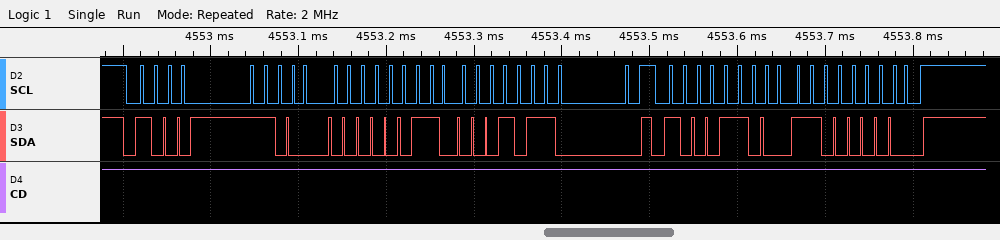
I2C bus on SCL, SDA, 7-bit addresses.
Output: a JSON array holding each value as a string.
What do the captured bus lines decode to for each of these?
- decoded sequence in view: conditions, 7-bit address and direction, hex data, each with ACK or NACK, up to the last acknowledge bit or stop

["start, address 46 write ACK, 03 ACK, 16 ACK, stop, start, address 46 write ACK, C0 ACK, stop"]
